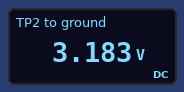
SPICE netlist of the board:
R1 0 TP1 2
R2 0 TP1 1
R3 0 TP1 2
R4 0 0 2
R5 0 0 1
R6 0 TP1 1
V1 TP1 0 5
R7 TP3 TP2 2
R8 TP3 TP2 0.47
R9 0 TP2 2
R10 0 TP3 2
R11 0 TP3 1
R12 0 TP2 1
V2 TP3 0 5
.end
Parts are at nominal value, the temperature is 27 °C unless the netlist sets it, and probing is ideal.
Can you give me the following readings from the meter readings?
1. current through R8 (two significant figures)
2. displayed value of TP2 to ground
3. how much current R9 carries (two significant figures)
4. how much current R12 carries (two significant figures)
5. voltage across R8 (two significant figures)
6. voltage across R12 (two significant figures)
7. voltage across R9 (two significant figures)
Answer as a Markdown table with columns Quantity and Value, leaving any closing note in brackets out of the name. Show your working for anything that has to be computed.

| Quantity | Value |
|---|---|
| current through R8 | (5 V - 3.183 V) / 470 mΩ = 3.9 A |
| displayed value of TP2 to ground | 3.183 V |
| how much current R9 carries | (3.183 V) / 2 Ω = 1.6 A |
| how much current R12 carries | (3.183 V) / 1 Ω = 3.2 A |
| voltage across R8 | 5 V - 3.183 V = 1.8 V |
| voltage across R12 | 3.183 V = 3.2 V |
| voltage across R9 | 3.183 V = 3.2 V |
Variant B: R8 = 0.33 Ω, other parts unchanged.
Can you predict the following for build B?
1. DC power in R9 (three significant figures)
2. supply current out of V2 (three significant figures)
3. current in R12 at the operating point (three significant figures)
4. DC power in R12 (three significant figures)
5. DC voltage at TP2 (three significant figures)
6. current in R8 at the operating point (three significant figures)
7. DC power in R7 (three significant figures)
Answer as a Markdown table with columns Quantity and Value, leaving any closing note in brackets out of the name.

| Quantity | Value |
|---|---|
| DC power in R9 | 6.16 W |
| supply current out of V2 | 12.8 A |
| current in R12 at the operating point | 3.51 A |
| DC power in R12 | 12.3 W |
| DC voltage at TP2 | 3.51 V |
| current in R8 at the operating point | 4.52 A |
| DC power in R7 | 1.11 W |
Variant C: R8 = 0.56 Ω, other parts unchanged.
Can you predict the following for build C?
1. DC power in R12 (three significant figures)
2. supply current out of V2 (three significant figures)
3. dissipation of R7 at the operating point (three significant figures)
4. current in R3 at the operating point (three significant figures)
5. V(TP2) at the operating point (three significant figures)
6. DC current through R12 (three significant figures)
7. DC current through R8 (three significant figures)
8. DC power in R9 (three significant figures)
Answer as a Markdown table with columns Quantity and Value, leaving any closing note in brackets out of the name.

| Quantity | Value |
|---|---|
| DC power in R12 | 9.11 W |
| supply current out of V2 | 12.0 A |
| dissipation of R7 at the operating point | 1.96 W |
| current in R3 at the operating point | 2.50 A |
| V(TP2) at the operating point | 3.02 V |
| DC current through R12 | 3.02 A |
| DC current through R8 | 3.54 A |
| DC power in R9 | 4.56 W |
